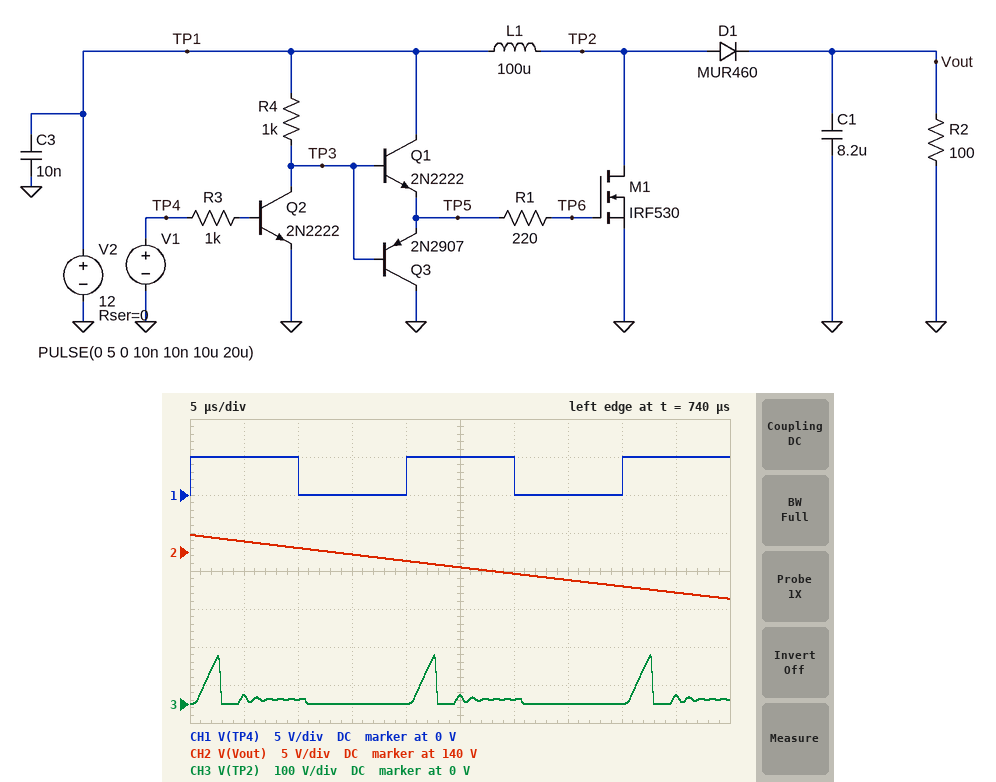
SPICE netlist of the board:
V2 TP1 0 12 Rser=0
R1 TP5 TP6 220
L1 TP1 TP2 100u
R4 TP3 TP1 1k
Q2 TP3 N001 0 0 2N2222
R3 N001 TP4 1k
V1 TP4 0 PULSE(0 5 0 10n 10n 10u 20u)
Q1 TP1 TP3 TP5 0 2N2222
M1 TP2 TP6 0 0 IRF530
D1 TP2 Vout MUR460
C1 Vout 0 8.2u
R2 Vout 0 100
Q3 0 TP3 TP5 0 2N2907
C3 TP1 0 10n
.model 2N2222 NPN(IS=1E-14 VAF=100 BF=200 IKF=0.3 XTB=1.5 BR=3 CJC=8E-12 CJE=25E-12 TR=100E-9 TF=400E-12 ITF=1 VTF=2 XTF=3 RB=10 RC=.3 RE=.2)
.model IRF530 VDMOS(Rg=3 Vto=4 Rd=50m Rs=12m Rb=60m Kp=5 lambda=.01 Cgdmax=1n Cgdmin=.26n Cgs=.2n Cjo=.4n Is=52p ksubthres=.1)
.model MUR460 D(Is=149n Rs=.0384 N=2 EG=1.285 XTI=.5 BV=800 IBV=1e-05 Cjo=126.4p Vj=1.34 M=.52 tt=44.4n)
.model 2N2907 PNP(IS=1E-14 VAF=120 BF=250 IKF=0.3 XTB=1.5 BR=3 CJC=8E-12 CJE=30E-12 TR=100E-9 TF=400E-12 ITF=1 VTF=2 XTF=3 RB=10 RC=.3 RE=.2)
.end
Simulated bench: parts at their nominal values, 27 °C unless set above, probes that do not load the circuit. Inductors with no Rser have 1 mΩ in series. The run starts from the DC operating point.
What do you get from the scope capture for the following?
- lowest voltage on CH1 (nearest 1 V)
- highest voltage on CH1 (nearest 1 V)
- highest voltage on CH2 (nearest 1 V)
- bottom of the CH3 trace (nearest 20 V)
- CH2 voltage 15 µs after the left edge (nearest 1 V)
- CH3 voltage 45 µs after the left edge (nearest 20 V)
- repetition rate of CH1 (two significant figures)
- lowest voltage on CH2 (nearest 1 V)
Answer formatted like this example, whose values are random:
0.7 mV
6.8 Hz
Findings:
0 V
5 V
142 V
0 V
140 V
20 V
50 kHz
134 V
